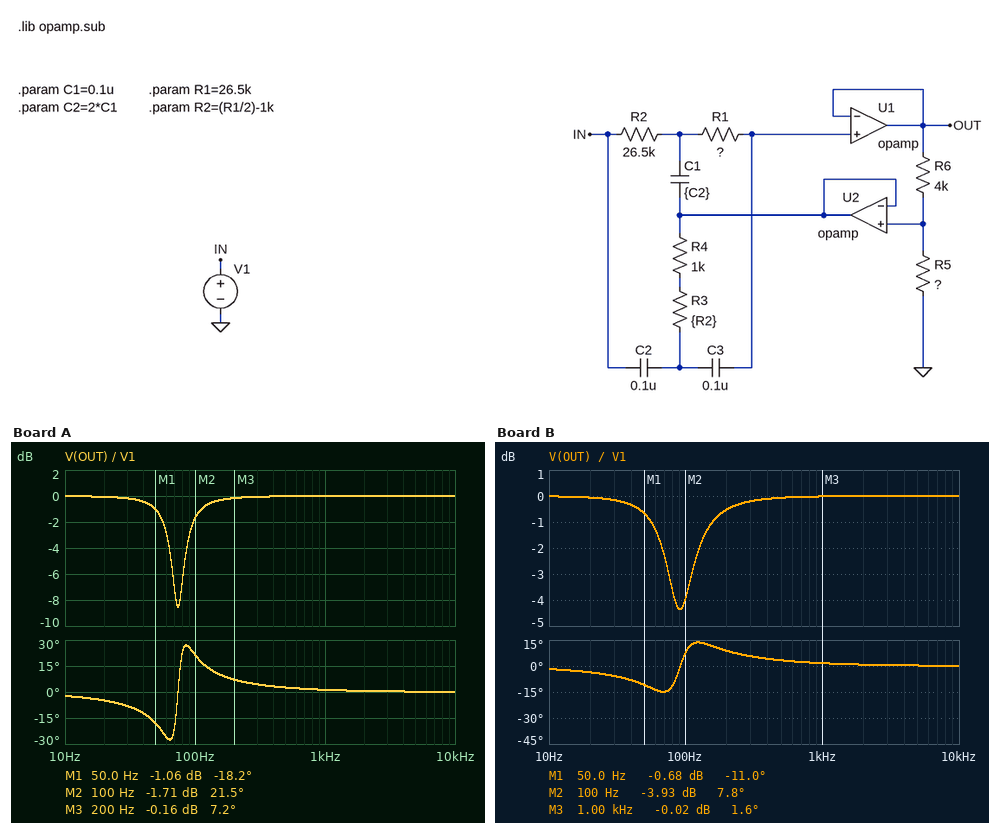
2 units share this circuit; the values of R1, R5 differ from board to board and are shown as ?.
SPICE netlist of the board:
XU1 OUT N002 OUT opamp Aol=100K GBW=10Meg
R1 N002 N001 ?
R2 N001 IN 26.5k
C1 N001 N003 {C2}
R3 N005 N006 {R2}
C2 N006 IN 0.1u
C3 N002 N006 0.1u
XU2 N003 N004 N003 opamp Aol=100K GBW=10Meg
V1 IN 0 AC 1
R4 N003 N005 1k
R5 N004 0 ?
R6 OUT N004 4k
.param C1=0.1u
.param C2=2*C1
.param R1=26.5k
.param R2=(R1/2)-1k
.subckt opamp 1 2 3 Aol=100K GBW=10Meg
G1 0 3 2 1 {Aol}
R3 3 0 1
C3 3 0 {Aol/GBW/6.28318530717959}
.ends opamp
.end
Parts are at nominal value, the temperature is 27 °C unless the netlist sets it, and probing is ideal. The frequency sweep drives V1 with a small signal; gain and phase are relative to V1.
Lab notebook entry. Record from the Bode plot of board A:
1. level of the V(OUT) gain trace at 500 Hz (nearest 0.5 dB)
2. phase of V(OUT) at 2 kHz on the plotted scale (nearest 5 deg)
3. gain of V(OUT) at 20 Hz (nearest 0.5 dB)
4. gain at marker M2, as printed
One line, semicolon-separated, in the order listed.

0 dB; 0 deg; 0 dB; -1.71 dB
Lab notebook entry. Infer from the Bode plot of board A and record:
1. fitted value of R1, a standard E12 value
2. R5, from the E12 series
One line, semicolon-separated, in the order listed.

15 kΩ; 56 kΩ
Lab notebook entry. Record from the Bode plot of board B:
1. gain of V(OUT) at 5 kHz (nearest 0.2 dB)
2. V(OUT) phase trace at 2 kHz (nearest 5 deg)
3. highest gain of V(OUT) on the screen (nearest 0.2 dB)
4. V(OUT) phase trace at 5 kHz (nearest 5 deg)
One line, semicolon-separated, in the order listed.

0 dB; 0 deg; 0 dB; 0 deg
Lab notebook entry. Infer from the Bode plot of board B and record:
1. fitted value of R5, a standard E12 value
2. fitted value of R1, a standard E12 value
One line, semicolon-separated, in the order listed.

68 kΩ; 8.2 kΩ
